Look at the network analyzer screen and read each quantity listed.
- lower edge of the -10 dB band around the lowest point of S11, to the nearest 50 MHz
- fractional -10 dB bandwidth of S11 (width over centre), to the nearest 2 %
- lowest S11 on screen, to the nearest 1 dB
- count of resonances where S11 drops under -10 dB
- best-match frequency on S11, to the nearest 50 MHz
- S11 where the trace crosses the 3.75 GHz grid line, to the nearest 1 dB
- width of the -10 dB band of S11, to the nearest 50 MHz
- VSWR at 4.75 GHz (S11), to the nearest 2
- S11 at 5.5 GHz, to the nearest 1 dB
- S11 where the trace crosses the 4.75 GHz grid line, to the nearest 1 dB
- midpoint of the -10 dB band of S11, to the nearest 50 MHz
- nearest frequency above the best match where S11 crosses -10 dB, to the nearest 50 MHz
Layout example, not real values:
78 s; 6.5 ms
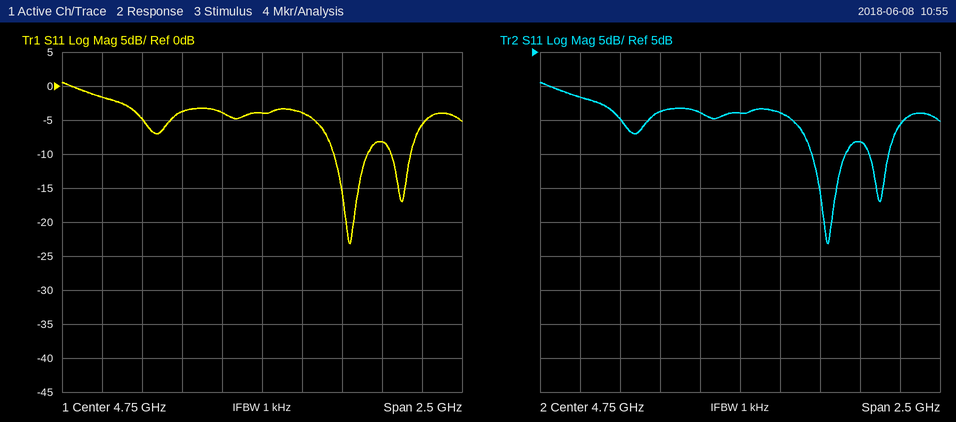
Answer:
5.20 GHz; 4 %; -23 dB; 2; 5.30 GHz; -2 dB; 200 MHz; 4; -8 dB; -4 dB; 5.30 GHz; 5.40 GHz
